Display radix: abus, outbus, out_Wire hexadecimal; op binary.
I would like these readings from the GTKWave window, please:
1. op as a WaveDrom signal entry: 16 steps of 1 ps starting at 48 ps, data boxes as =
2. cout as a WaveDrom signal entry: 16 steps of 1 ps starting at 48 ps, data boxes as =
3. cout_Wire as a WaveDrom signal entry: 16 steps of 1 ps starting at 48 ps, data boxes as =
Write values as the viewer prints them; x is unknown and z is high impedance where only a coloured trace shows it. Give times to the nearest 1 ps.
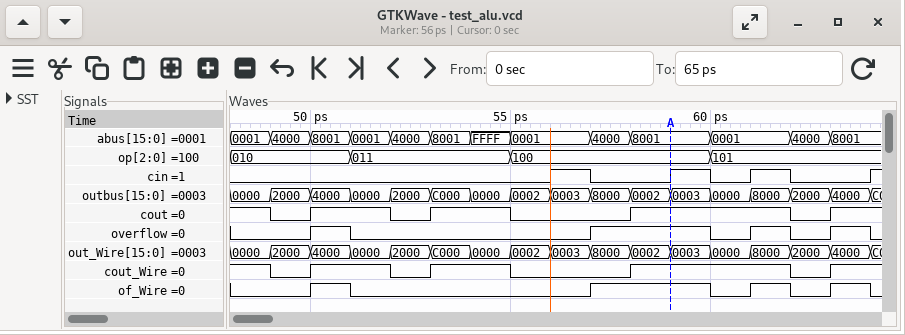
{name: 'op', wave: '=..=...=....=...', data: '010 011 100 101'}
{name: 'cout', wave: '101.01.0..1...01'}
{name: 'cout_Wire', wave: '101.01.0..1...01'}
